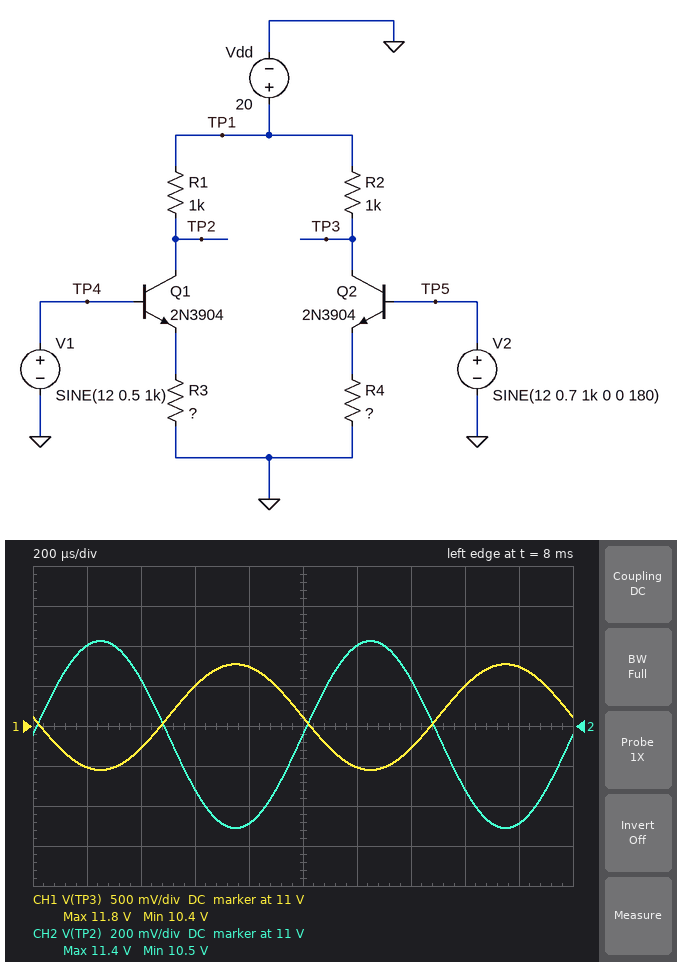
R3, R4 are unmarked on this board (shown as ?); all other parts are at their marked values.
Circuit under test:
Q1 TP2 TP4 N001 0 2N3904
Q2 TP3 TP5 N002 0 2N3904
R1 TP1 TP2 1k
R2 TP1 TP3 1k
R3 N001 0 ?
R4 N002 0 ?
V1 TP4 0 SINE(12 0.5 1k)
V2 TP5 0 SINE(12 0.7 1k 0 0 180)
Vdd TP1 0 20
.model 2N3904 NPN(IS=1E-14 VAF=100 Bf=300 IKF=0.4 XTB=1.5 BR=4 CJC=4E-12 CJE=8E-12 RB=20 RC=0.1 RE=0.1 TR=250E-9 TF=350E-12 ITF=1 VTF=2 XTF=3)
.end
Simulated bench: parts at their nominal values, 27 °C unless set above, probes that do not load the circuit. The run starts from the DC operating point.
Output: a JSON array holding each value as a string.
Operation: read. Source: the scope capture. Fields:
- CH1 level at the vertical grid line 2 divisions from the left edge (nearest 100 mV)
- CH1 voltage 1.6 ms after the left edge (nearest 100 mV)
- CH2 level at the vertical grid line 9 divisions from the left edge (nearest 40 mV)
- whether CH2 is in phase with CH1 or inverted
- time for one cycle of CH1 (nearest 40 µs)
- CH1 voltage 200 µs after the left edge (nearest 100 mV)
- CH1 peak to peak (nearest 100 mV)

["10.7 V", "11.5 V", "10.52 V", "inverted", "1.00 ms", "10.5 V", "1.3 V"]
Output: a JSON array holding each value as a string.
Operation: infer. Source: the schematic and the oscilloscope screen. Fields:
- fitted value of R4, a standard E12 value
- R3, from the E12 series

["680 Ω", "470 Ω"]
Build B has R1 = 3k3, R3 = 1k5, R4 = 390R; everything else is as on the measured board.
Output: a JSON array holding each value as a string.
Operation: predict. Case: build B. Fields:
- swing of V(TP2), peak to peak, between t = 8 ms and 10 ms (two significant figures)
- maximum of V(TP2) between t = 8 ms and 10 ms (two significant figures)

["980 mV", "12 V"]
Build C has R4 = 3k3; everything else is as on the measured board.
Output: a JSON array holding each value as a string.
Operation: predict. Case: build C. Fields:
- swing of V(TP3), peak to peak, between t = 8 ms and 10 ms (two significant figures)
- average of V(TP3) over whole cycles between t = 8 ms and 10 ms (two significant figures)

["420 mV", "17 V"]
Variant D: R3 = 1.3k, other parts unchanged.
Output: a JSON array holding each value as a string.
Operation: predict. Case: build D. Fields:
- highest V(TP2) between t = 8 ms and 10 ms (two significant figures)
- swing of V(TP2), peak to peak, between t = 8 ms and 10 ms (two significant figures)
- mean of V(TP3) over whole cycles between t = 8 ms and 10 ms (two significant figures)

["12 V", "410 mV", "11 V"]
